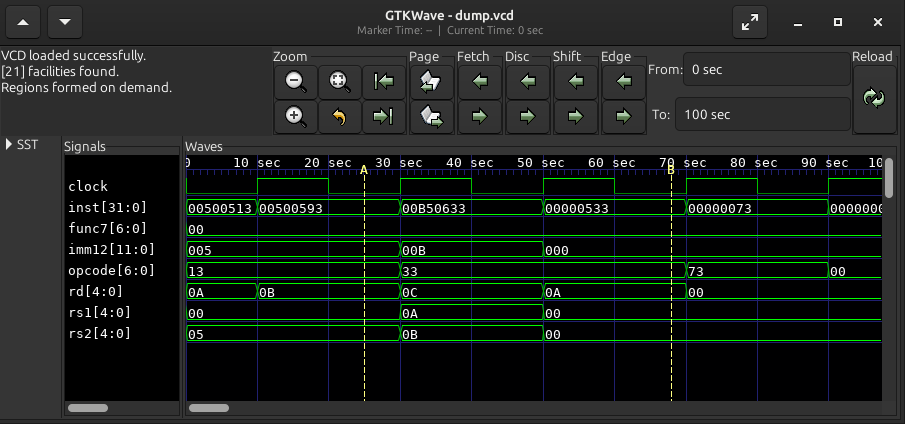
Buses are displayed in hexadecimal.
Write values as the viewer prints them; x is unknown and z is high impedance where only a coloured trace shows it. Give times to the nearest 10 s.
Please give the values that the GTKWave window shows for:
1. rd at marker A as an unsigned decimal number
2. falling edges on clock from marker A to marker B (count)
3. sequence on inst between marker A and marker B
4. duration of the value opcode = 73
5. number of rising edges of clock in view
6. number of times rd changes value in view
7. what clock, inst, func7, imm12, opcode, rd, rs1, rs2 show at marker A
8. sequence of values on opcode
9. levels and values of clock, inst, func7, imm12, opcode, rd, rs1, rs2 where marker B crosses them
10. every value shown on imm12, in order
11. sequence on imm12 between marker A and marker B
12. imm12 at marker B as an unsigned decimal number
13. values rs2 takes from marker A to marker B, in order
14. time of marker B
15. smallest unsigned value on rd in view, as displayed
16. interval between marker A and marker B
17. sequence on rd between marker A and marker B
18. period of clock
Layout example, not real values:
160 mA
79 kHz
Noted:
11
2
00500593, 00B50633, 00000533
20 s
5
4
clock=0, inst=00500593, func7=00, imm12=005, opcode=13, rd=0B, rs1=00, rs2=05
13, 33, 73, 00
clock=0, inst=00000533, func7=00, imm12=000, opcode=33, rd=0A, rs1=00, rs2=00
005, 00B, 000
005, 00B, 000
0
05, 0B, 00
70 s
00
40 s
0B, 0C, 0A
20 s
